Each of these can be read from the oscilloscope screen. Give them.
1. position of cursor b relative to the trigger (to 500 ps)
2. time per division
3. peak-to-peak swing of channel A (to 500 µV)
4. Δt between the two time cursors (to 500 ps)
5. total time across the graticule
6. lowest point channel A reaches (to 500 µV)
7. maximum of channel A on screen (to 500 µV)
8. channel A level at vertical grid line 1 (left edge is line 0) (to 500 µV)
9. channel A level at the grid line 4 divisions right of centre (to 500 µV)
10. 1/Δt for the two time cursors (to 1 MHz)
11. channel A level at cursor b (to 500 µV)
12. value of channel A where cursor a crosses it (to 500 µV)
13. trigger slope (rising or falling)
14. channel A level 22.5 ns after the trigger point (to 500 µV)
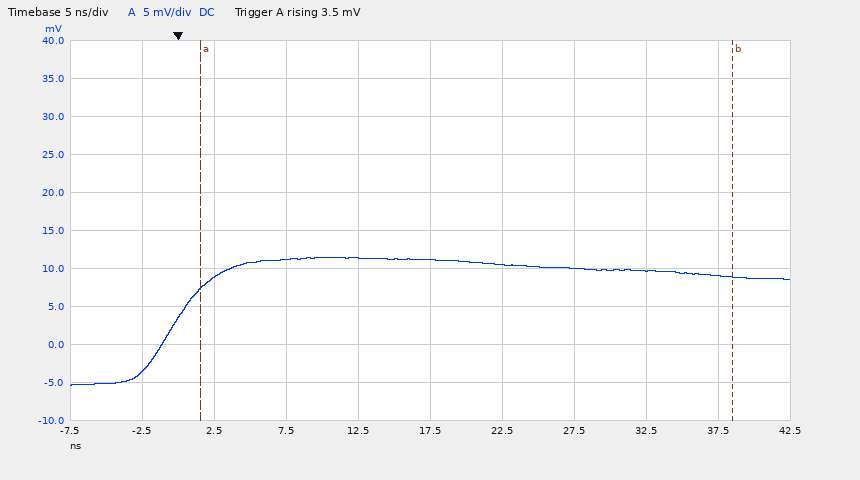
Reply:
+38.5 ns
5 ns
17.0 mV
37.0 ns
50 ns
-5.5 mV
11.5 mV
-3.5 mV
9.0 mV
27 MHz
9.0 mV
7.5 mV
rising
10.5 mV
